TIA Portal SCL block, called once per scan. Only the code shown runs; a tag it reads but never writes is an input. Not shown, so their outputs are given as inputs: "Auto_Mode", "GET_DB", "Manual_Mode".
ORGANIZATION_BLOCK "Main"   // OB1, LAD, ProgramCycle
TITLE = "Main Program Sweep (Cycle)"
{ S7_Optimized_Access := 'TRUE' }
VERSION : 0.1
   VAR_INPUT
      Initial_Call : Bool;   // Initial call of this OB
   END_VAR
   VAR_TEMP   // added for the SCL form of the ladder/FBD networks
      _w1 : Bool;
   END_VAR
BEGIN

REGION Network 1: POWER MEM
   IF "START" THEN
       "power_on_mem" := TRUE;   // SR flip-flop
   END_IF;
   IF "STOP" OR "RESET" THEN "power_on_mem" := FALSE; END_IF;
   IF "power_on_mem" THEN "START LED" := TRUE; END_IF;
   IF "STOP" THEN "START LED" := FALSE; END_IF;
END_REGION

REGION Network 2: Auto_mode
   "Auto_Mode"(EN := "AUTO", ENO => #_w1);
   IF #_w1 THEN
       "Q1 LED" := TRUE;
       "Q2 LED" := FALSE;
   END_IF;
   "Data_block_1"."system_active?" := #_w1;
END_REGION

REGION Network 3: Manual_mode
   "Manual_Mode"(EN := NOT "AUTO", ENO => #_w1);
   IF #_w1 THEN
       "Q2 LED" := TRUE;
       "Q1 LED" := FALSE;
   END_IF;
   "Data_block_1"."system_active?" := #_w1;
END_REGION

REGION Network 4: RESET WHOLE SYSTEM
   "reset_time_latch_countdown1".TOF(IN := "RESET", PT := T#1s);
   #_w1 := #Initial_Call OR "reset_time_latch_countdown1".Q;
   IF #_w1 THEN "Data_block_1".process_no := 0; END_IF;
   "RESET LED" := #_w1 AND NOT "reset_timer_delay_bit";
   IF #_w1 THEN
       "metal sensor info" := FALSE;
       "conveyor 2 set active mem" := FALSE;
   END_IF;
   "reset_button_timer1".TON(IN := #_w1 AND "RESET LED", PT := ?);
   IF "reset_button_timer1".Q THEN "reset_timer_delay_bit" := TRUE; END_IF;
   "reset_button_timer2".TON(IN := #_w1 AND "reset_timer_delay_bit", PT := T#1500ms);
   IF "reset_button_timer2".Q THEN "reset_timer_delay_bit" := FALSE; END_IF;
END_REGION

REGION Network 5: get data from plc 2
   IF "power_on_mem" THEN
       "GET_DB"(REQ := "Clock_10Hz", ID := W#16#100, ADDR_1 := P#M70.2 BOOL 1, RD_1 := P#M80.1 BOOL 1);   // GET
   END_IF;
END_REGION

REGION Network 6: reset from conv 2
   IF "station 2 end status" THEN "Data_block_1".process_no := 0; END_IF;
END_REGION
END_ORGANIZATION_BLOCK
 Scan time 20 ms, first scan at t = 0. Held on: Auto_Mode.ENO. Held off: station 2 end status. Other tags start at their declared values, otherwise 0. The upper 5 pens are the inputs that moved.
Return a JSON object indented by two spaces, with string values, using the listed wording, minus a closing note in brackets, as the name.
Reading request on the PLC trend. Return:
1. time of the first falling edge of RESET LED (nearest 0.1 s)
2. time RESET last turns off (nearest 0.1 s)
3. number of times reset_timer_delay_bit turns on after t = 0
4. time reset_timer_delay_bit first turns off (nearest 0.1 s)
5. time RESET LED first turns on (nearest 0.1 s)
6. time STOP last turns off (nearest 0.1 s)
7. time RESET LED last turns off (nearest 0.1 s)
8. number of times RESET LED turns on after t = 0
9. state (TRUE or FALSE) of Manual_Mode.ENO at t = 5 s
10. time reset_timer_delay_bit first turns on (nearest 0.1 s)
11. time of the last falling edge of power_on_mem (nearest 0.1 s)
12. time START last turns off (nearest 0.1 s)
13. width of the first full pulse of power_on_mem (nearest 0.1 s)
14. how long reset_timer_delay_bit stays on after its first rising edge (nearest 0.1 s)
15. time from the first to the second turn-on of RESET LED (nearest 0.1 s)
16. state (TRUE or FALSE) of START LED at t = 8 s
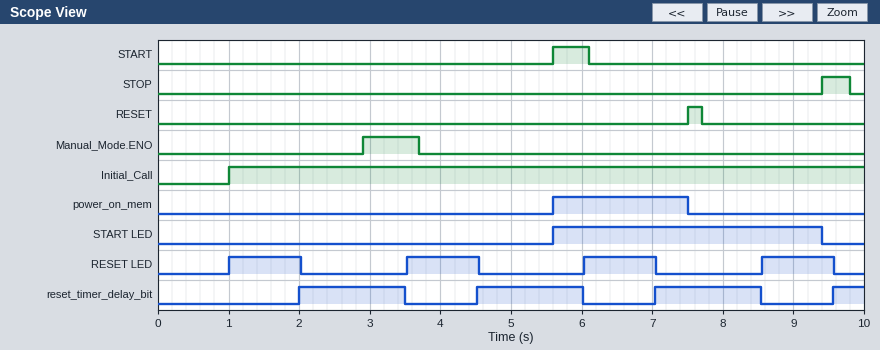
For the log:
{
  "time of the first falling edge of RESET LED": "2.0 s",
  "time RESET last turns off": "7.7 s",
  "number of times reset_timer_delay_bit turns on after t = 0": "4",
  "time reset_timer_delay_bit first turns off": "3.5 s",
  "time RESET LED first turns on": "1.0 s",
  "time STOP last turns off": "9.8 s",
  "time RESET LED last turns off": "9.6 s",
  "number of times RESET LED turns on after t = 0": "4",
  "state (TRUE or FALSE) of Manual_Mode.ENO at t = 5 s": "FALSE",
  "time reset_timer_delay_bit first turns on": "2.0 s",
  "time of the last falling edge of power_on_mem": "7.5 s",
  "time START last turns off": "6.1 s",
  "width of the first full pulse of power_on_mem": "1.9 s",
  "how long reset_timer_delay_bit stays on after its first rising edge": "1.5 s",
  "time from the first to the second turn-on of RESET LED": "2.5 s",
  "state (TRUE or FALSE) of START LED at t = 8 s": "TRUE"
}
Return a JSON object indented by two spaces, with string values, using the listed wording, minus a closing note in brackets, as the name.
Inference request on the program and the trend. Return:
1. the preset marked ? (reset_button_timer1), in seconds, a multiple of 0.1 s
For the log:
{
  "the preset marked ? (reset_button_timer1), in seconds, a multiple of 0.1 s": "1.0 s"
}
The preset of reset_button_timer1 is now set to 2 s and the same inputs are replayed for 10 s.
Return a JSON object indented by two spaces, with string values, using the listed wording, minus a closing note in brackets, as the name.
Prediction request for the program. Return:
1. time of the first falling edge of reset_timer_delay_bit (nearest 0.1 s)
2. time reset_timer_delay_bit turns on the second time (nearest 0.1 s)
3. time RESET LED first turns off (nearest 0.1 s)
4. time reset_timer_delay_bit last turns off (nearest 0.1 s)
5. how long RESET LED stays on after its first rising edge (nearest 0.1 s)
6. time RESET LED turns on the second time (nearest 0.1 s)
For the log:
{
  "time of the first falling edge of reset_timer_delay_bit": "4.5 s",
  "time reset_timer_delay_bit turns on the second time": "6.5 s",
  "time RESET LED first turns off": "3.0 s",
  "time reset_timer_delay_bit last turns off": "8.0 s",
  "how long RESET LED stays on after its first rising edge": "2.0 s",
  "time RESET LED turns on the second time": "4.5 s"
}
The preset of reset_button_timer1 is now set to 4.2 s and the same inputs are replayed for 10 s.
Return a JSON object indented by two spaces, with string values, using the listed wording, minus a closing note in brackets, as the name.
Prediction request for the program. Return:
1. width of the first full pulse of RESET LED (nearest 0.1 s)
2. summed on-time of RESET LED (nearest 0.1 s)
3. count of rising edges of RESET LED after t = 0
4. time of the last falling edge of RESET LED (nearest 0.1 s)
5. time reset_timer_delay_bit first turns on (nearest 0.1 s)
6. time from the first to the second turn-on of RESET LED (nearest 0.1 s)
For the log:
{
  "width of the first full pulse of RESET LED": "4.2 s",
  "summed on-time of RESET LED": "7.5 s",
  "count of rising edges of RESET LED after t = 0": "2",
  "time of the last falling edge of RESET LED": "5.2 s",
  "time reset_timer_delay_bit first turns on": "5.2 s",
  "time from the first to the second turn-on of RESET LED": "5.7 s"
}
